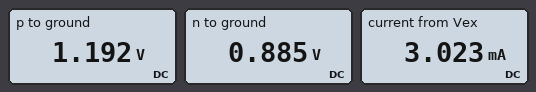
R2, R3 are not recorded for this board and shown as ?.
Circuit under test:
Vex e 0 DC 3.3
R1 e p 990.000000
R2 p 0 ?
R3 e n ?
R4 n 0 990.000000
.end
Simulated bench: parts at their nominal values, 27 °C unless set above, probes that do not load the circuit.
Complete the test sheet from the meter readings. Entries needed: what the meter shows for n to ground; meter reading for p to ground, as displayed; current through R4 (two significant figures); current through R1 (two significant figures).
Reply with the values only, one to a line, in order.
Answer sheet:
0.885 V
1.192 V
890 µA
2.1 mA
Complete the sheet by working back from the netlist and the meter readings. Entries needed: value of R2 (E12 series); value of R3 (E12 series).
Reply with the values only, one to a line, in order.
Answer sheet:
560 Ω
2.7 kΩ
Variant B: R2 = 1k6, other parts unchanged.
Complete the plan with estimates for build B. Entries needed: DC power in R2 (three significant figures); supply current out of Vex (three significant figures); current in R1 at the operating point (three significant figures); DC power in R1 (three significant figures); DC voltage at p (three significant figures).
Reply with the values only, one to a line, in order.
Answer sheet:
2.60 mW
2.17 mA
1.27 mA
1.61 mW
2.04 V
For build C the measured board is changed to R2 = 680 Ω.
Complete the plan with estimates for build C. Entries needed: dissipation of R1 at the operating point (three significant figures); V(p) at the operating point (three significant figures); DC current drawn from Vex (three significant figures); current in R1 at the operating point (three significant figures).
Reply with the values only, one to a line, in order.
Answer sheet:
3.87 mW
1.34 V
2.87 mA
1.98 mA
